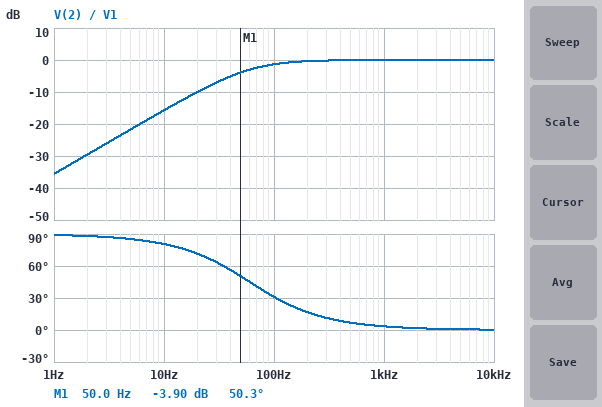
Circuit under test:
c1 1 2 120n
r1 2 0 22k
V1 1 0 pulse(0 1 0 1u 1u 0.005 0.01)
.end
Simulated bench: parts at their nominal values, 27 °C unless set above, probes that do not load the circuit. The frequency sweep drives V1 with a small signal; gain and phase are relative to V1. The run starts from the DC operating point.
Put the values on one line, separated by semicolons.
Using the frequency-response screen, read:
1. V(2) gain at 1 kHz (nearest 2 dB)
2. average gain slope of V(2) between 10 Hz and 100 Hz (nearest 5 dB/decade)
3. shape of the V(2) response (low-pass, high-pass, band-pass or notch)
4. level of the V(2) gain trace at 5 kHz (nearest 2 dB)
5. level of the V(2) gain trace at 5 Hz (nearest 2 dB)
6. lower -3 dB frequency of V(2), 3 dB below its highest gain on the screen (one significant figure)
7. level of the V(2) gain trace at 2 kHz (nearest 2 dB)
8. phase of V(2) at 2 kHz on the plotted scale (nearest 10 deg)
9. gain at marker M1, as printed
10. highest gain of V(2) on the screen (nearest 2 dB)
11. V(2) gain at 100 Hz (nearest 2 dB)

0 dB; 15 dB/decade; high-pass; 0 dB; -22 dB; 60 Hz; 0 dB; 0 deg; -3.90 dB; 0 dB; -2 dB
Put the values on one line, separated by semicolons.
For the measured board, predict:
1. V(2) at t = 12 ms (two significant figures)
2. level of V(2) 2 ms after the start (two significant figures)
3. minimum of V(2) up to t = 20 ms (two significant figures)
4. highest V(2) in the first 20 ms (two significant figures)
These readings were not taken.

410 mV; 470 mV; -870 mV; 1.0 V
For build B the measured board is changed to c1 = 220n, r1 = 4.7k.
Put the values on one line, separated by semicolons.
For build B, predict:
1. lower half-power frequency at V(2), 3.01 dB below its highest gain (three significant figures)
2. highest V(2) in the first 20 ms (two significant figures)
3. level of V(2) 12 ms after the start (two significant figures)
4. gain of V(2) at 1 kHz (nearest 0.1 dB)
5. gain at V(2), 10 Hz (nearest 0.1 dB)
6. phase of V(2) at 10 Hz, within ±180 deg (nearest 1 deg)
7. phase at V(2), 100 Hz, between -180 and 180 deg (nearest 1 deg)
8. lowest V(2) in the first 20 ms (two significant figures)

154 Hz; 1.0 V; 140 mV; -0.1 dB; -23.8 dB; 86 deg; 57 deg; -990 mV
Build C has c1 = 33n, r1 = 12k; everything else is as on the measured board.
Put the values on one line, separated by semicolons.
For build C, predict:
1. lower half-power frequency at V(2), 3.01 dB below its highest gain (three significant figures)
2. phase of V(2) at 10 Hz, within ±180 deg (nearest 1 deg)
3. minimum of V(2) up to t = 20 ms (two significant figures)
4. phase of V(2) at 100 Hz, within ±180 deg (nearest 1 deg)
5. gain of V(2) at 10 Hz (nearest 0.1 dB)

402 Hz; 89 deg; -1.0 V; 76 deg; -32.1 dB
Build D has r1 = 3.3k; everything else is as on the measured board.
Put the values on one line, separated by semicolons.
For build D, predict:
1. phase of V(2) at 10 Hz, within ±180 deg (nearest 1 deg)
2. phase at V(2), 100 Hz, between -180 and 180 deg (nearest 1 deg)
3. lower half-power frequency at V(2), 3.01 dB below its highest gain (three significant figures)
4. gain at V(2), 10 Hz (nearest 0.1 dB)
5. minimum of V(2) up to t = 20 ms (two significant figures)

89 deg; 76 deg; 402 Hz; -32.1 dB; -1.0 V
